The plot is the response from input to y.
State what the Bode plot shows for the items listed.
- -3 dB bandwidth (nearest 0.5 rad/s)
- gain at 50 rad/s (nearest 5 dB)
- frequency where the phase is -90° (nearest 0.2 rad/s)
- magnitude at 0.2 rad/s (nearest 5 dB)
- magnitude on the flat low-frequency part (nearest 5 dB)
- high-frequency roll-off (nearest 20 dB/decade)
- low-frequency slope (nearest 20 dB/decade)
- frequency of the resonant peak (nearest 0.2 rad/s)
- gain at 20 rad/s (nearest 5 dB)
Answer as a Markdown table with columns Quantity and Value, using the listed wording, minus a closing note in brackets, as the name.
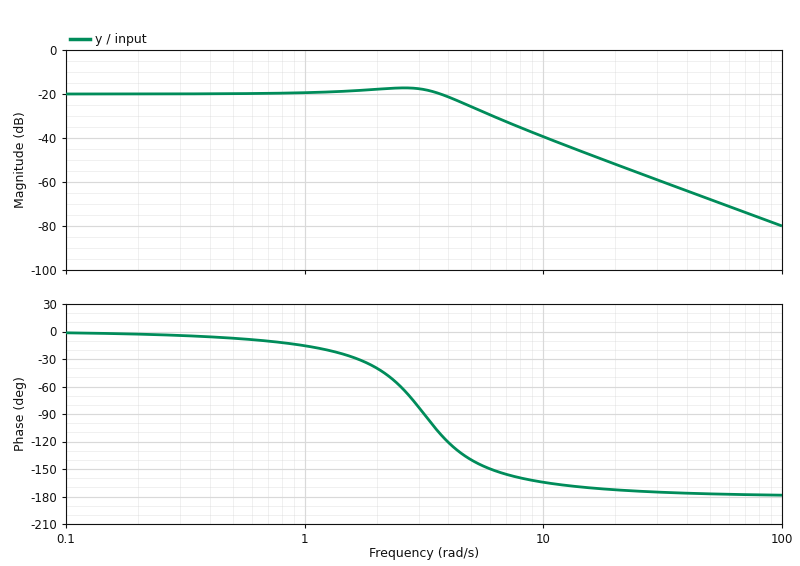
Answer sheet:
| Quantity | Value |
|---|---|
| -3 dB bandwidth | 4.5 rad/s |
| gain at 50 rad/s | -70 dB |
| frequency where the phase is -90° | 3.2 rad/s |
| magnitude at 0.2 rad/s | -20 dB |
| magnitude on the flat low-frequency part | -20 dB |
| high-frequency roll-off | -40 dB/decade |
| low-frequency slope | 0 dB/decade |
| frequency of the resonant peak | 2.6 rad/s |
| gain at 20 rad/s | -50 dB |
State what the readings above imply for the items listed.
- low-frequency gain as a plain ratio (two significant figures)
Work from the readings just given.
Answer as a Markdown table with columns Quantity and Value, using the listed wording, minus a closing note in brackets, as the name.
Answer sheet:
| Quantity | Value |
|---|---|
| low-frequency gain as a plain ratio | 0.10 |
